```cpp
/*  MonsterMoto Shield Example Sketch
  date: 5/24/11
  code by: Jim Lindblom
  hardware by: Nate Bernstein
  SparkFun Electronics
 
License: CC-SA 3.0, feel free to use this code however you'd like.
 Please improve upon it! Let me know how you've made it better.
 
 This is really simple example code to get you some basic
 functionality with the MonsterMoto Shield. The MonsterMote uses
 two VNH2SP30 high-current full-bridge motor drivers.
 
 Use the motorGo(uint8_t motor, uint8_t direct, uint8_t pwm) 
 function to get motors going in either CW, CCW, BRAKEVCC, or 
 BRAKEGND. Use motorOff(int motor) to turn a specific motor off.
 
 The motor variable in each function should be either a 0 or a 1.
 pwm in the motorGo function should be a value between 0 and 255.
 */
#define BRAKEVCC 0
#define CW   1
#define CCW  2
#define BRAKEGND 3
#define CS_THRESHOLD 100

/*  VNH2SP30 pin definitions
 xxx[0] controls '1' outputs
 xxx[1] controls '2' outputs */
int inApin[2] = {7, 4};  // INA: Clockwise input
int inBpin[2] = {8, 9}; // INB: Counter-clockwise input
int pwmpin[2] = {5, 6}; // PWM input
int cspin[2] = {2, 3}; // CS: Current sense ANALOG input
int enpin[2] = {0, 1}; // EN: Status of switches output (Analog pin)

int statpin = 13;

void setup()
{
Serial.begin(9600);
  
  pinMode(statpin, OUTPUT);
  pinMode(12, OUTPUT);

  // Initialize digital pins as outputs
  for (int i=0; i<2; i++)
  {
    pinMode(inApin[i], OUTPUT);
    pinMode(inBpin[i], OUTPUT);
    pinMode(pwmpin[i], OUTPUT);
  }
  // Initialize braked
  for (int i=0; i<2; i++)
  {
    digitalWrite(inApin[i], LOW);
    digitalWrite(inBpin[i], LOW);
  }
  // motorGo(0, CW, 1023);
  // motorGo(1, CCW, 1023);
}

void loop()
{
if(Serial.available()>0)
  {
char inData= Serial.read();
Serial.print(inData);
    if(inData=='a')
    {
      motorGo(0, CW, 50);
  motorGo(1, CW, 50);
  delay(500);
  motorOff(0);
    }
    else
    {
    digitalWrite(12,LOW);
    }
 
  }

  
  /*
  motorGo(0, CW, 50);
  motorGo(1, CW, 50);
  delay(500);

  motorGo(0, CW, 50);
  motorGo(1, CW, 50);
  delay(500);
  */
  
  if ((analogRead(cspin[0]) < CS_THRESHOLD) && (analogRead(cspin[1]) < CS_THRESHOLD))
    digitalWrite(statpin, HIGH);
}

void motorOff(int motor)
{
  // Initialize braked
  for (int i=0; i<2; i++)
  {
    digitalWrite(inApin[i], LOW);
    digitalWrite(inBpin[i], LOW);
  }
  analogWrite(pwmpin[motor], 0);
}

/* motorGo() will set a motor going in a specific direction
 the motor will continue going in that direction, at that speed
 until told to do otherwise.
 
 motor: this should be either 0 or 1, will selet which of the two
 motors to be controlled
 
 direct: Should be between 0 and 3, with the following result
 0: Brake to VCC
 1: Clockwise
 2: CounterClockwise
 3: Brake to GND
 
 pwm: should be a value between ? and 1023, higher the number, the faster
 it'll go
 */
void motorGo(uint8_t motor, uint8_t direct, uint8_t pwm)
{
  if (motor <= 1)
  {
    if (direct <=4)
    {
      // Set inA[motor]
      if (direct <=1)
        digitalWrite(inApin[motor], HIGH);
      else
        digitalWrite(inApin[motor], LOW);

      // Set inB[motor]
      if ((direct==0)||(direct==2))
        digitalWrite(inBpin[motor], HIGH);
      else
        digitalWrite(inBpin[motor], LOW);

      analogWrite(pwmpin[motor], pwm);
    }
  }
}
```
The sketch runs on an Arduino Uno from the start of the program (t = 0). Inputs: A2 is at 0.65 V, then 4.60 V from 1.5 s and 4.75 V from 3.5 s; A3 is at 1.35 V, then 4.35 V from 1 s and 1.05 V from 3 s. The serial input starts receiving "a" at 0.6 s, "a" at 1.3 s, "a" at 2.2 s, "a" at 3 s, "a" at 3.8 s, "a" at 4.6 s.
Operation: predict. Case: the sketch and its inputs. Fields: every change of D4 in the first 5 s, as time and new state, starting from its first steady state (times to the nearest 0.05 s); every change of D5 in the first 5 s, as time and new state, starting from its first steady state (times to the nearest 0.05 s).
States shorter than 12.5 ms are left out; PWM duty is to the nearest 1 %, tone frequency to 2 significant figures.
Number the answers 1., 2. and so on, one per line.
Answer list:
1. 0 s low; 0.6 s high; 1.1 s low; 1.3 s high; 1.8 s low; 2.2 s high; 2.7 s low; 3 s high; 3.5 s low; 3.8 s high; 4.3 s low; 4.6 s high
2. 0 s low; 0.6 s PWM 20 %; 1.1 s low; 1.3 s PWM 20 %; 1.8 s low; 2.2 s PWM 20 %; 2.7 s low; 3 s PWM 20 %; 3.5 s low; 3.8 s PWM 20 %; 4.3 s low; 4.6 s PWM 20 %
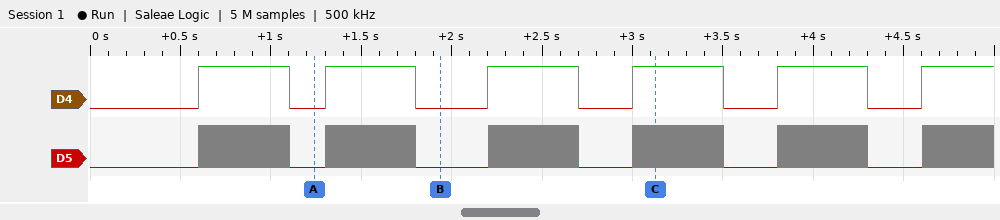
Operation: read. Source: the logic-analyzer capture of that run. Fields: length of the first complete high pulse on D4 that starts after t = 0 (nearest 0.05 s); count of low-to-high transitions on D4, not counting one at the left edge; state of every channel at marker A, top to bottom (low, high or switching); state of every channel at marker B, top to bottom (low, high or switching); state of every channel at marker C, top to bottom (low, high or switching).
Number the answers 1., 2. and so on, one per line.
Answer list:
1. 0.50 s
2. 6
3. D4 low, D5 low
4. D4 low, D5 low
5. D4 high, D5 switching
